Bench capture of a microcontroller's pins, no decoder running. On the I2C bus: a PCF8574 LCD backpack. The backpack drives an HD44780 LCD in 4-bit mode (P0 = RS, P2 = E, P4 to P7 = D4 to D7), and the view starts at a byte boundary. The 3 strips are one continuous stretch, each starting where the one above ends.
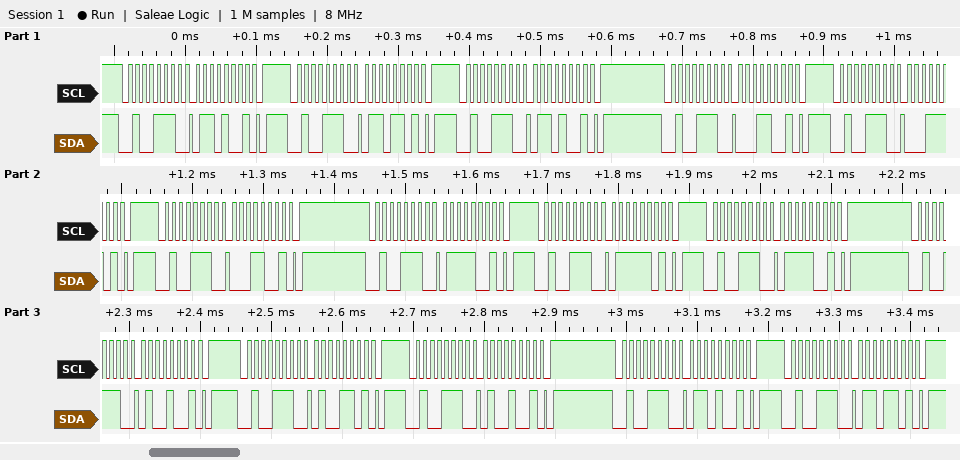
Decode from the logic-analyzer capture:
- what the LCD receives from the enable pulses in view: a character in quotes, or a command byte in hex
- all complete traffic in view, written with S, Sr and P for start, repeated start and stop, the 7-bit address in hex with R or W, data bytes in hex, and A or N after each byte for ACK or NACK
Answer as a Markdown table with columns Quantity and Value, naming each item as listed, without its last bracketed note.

| Quantity | Value |
|---|---|
| what the LCD receives from the enable pulses in view: a character in quotes, or a command byte in hex | 'a' 't' |
| all complete traffic in view, written with S, Sr and P for start, repeated start and stop, the 7-bit address in hex with R or W, data bytes in hex, and A or N after each byte for ACK or NACK | S 27W A 69 A P S 27W A 6D A P S 27W A 69 A P S 27W A 19 A P S 27W A 1D A P S 27W A 19 A P S 27W A 79 A P S 27W A 7D A P S 27W A 79 A P S 27W A 49 A P S 27W A 4D A P S 27W A 49 A P S 27W A 69 A P S 27W A 6D A P |
